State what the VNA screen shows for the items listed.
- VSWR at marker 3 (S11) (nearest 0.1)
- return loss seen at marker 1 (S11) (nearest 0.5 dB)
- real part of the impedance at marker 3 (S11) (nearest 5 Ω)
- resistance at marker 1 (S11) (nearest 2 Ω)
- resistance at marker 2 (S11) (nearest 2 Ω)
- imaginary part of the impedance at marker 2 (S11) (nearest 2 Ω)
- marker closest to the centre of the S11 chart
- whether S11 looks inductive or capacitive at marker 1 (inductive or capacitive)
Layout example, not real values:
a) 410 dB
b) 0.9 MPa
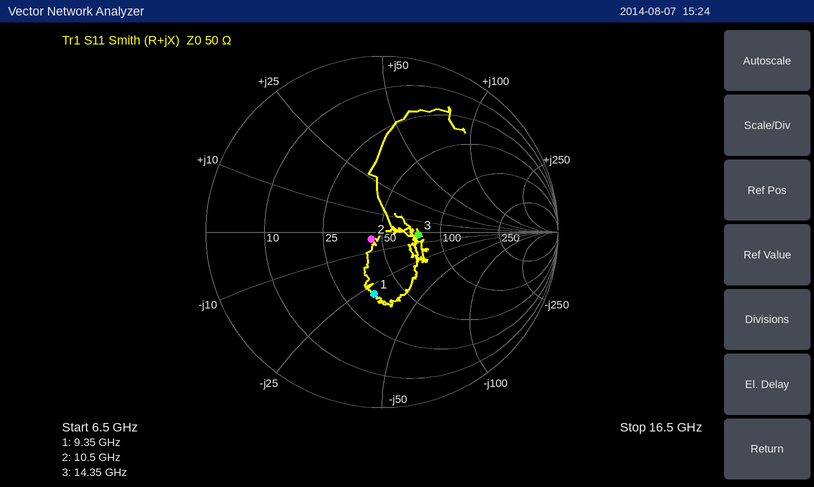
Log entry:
a) 1.5
b) 9.0 dB
c) 75 Ω
d) 36 Ω
e) 44 Ω
f) -4 Ω
g) marker 2
h) capacitive
